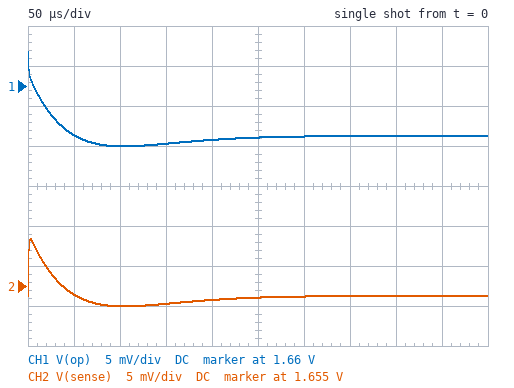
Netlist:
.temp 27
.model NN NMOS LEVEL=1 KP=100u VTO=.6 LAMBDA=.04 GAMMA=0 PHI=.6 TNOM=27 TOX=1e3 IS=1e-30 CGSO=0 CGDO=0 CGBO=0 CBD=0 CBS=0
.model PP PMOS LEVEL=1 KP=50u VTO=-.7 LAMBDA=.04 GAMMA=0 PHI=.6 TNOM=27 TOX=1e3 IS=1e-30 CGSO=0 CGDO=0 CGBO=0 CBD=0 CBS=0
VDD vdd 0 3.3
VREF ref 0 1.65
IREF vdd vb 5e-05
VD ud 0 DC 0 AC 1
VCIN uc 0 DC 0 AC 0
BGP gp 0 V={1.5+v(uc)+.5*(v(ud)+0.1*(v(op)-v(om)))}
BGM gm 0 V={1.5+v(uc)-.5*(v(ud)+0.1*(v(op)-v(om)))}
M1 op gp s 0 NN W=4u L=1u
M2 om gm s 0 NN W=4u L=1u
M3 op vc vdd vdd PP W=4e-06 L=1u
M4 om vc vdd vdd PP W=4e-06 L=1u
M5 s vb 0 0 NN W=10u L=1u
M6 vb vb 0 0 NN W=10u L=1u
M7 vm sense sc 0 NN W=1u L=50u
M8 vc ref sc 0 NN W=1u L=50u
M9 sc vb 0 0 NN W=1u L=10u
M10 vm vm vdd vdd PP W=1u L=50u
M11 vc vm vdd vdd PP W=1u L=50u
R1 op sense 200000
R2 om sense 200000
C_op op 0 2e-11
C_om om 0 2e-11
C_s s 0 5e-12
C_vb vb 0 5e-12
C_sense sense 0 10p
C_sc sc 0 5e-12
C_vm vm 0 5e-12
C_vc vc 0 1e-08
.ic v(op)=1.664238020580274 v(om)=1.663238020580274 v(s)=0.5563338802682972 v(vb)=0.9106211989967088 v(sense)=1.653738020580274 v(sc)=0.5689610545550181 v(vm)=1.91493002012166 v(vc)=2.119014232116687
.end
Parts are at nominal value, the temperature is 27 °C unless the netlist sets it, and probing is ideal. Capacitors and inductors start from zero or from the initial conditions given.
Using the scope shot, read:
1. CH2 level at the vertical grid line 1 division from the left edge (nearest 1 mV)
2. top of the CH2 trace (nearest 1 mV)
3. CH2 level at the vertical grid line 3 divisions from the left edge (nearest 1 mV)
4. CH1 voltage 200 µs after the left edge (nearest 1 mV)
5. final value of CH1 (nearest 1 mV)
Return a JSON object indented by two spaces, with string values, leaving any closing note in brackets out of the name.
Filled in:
{
  "CH2 level at the vertical grid line 1 division from the left edge": "1.654 V",
  "top of the CH2 trace": "1.661 V",
  "CH2 level at the vertical grid line 3 divisions from the left edge": "1.653 V",
  "CH1 voltage 200 µs after the left edge": "1.653 V",
  "final value of CH1": "1.654 V"
}
